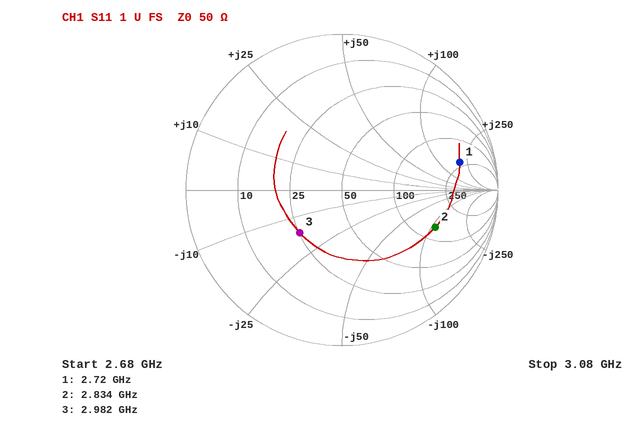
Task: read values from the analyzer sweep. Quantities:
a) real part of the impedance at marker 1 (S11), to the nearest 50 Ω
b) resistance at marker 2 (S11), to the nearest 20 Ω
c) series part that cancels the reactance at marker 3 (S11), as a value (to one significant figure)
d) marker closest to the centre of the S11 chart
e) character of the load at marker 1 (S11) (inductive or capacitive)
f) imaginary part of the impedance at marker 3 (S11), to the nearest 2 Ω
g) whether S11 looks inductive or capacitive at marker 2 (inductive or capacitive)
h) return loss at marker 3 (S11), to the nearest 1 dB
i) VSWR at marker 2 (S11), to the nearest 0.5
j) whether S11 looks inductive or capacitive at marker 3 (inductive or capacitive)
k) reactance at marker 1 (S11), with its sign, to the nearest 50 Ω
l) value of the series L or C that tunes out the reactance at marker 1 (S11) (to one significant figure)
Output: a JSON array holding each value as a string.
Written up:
["200 Ω", "140 Ω", "900 pH", "marker 3", "inductive", "-16 Ω", "capacitive", "8 dB", "4.5", "capacitive", "+200 Ω", "300 fF"]
